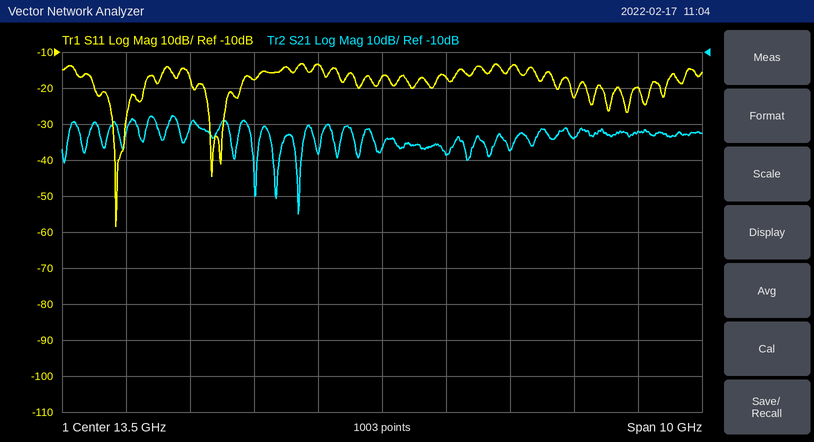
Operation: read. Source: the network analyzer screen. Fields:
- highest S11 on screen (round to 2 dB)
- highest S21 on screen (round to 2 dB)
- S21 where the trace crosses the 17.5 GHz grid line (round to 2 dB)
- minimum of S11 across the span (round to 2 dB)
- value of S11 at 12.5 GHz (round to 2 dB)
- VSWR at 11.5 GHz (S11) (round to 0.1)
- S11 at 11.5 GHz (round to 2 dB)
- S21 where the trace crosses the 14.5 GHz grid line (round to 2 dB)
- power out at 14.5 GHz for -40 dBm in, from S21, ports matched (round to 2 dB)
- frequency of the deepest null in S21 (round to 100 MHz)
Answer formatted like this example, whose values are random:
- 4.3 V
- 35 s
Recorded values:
- -14 dB
- -28 dB
- -32 dB
- -58 dB
- -14 dB
- 1.3
- -18 dB
- -38 dB
- -78 dBm
- 12.2 GHz
